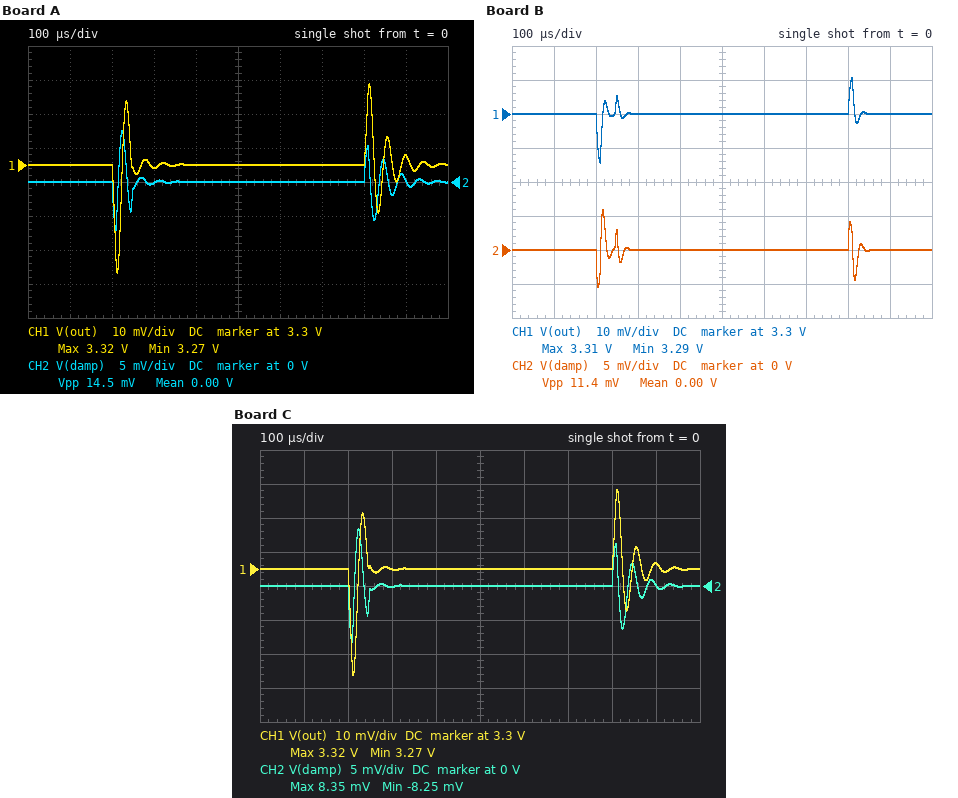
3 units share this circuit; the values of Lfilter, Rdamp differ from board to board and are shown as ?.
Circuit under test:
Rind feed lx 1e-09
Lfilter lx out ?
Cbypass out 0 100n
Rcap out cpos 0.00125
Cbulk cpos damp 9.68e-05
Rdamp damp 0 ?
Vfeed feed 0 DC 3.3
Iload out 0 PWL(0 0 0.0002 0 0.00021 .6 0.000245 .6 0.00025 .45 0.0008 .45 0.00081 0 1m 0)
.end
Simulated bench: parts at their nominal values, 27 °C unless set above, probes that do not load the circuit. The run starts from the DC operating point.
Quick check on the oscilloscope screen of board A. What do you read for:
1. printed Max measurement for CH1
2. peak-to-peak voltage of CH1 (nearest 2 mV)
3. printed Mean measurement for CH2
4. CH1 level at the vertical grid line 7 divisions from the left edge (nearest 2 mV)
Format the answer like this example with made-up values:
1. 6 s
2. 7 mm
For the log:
1. 3.32 V
2. 56 mV
3. 0.00 V
4. 3.300 V
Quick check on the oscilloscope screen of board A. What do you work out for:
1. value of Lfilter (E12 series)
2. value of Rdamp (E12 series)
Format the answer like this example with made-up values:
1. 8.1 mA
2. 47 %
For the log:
1. 470 nH
2. 0.022 Ω
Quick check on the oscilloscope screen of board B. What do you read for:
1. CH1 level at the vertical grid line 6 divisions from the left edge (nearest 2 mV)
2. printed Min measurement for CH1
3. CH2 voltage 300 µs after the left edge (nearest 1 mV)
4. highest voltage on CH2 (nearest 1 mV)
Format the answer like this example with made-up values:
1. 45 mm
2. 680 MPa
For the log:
1. 3.300 V
2. 3.29 V
3. 0 V
4. 6 mV
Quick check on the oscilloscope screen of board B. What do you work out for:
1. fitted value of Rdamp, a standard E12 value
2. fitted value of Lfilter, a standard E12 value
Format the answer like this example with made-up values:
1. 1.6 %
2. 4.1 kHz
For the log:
1. 0.039 Ω
2. 180 nH
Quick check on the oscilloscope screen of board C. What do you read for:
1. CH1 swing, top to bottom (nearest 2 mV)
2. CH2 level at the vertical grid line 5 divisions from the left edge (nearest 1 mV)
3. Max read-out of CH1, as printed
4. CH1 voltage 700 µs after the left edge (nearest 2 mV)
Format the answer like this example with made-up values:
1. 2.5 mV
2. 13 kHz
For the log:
1. 54 mV
2. 0 V
3. 3.32 V
4. 3.300 V
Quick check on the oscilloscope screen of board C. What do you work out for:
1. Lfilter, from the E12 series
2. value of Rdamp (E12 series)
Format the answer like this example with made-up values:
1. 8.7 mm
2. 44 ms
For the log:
1. 470 nH
2. 0.027 Ω
